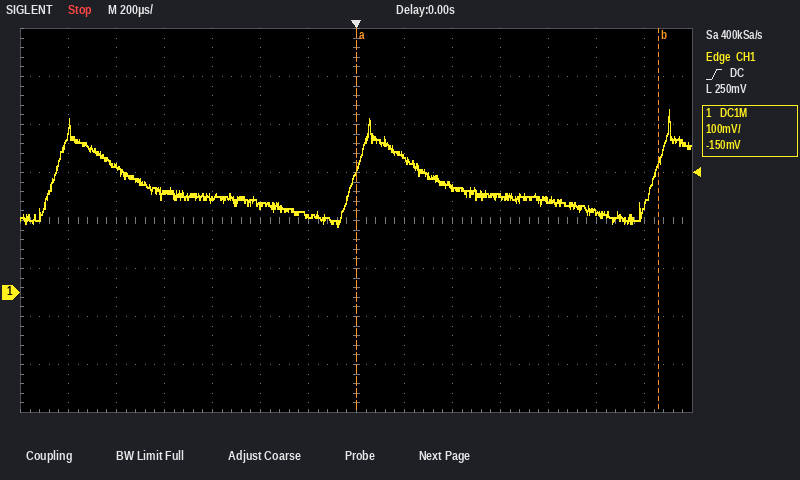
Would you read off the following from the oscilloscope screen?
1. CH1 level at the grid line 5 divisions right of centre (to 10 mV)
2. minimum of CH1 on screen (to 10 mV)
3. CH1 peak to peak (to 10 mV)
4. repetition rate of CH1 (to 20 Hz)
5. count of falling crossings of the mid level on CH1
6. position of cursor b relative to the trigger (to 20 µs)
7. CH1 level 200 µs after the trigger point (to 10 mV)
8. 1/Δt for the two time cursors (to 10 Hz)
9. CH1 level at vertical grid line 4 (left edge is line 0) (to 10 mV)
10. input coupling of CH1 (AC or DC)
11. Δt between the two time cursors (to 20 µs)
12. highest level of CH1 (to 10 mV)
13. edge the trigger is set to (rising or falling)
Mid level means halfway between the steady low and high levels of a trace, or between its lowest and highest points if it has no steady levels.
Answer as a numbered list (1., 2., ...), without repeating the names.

1. 170 mV
2. 140 mV
3. 240 mV
4. 800 Hz
5. 2
6. +1.26 ms
7. 280 mV
8. 790 Hz
9. 190 mV
10. DC
11. 1.26 ms
12. 380 mV
13. rising
